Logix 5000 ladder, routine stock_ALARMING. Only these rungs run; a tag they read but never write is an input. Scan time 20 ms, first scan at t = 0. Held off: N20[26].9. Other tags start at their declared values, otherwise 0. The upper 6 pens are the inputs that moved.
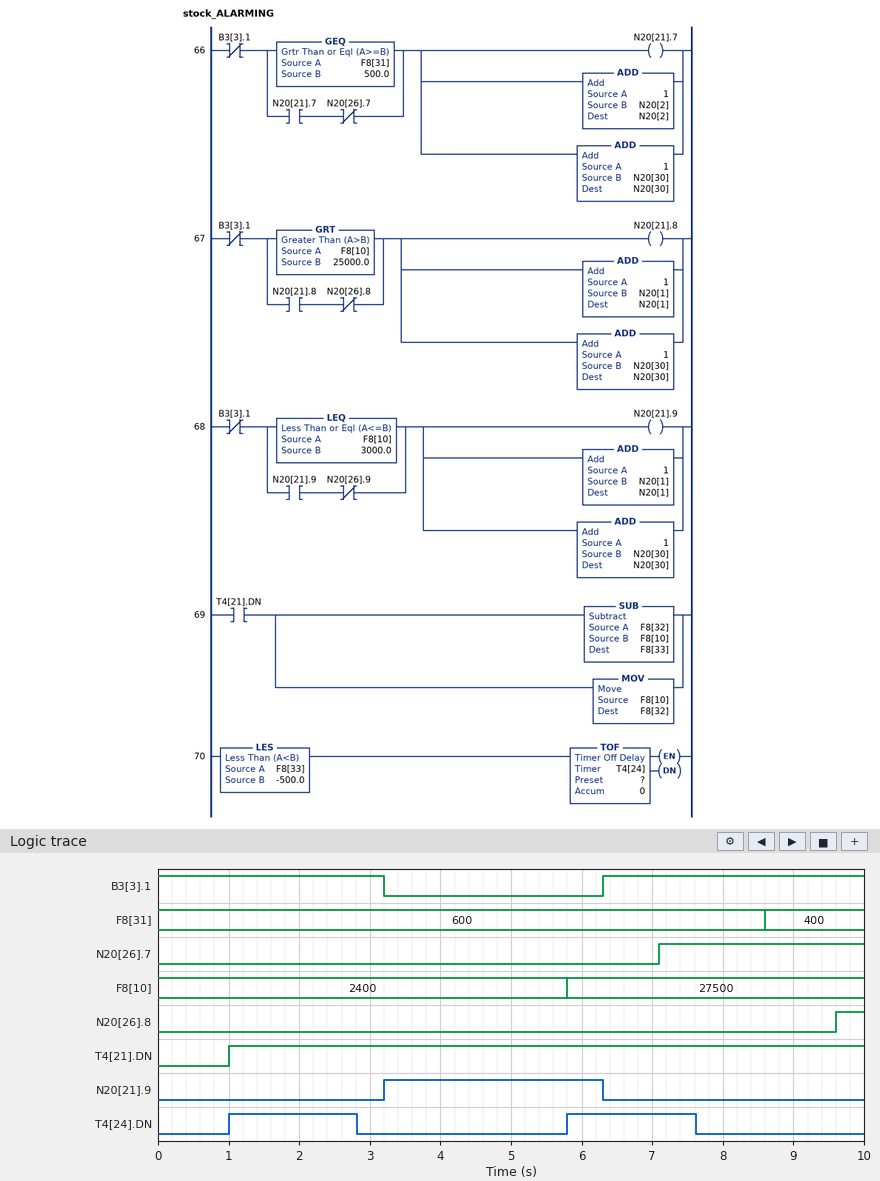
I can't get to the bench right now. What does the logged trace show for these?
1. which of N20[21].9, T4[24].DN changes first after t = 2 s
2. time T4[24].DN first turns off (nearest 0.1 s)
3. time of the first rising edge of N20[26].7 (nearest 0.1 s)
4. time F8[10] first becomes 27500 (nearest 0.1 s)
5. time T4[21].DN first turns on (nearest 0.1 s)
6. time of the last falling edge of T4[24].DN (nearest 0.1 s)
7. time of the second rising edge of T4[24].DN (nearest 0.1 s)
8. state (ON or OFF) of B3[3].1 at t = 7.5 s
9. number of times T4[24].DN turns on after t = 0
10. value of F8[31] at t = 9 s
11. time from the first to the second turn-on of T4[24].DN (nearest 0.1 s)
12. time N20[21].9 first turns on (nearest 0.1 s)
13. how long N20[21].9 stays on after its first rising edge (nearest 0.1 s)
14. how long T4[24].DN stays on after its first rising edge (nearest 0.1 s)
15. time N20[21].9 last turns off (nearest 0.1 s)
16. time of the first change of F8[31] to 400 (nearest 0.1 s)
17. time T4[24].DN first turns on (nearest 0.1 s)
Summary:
T4[24].DN
2.8 s
7.1 s
5.8 s
1.0 s
7.6 s
5.8 s
ON
2
400
4.8 s
3.2 s
3.1 s
1.8 s
6.3 s
8.6 s
1.0 s
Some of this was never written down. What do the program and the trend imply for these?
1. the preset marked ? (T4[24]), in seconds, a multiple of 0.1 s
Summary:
1.8 s
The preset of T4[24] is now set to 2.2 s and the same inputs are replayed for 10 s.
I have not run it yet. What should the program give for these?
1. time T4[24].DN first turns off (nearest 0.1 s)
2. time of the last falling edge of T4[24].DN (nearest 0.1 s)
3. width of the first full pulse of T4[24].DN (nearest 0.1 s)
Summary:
3.2 s
8.0 s
2.2 s
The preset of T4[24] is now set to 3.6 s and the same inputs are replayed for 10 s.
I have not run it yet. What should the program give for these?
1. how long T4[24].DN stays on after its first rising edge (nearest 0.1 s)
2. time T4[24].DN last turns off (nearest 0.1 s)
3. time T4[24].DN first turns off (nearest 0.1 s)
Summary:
3.6 s
9.4 s
4.6 s
